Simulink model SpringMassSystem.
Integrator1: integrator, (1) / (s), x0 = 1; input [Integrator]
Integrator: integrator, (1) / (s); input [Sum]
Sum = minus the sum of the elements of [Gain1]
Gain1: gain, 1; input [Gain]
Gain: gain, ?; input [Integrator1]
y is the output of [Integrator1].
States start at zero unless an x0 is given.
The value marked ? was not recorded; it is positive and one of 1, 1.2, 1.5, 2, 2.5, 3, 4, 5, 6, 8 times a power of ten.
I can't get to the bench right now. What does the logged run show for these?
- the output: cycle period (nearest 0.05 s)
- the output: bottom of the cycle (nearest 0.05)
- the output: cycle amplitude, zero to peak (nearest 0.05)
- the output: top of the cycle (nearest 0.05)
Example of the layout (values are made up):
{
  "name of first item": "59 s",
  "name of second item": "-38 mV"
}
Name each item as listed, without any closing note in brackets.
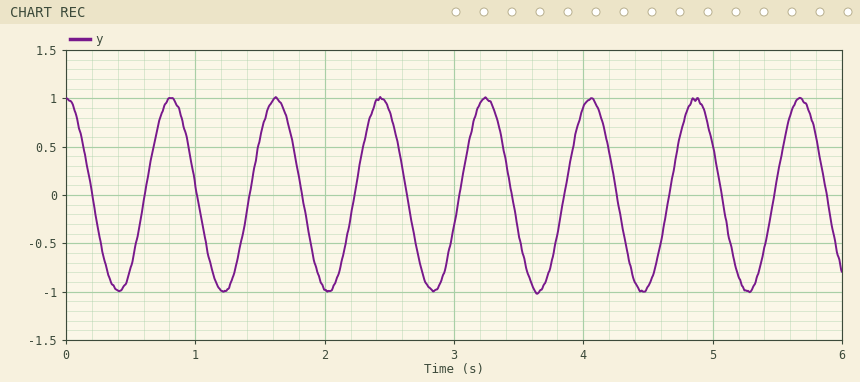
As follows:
{
  "the output: cycle period": "0.80 s",
  "the output: bottom of the cycle": "-1.00",
  "the output: cycle amplitude, zero to peak": "1.00",
  "the output: top of the cycle": "1.00"
}
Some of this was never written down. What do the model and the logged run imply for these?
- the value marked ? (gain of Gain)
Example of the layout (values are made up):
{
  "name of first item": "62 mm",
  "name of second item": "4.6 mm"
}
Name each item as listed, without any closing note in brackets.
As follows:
{
  "the value marked ?": "60"
}
